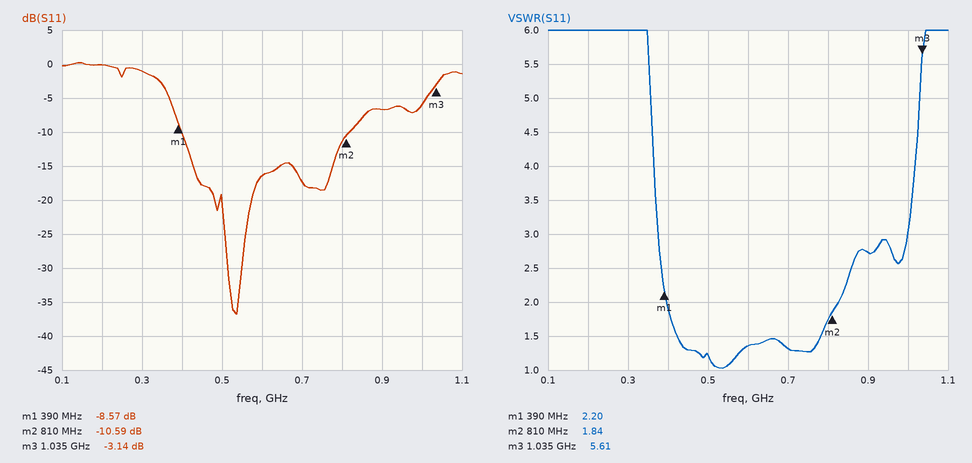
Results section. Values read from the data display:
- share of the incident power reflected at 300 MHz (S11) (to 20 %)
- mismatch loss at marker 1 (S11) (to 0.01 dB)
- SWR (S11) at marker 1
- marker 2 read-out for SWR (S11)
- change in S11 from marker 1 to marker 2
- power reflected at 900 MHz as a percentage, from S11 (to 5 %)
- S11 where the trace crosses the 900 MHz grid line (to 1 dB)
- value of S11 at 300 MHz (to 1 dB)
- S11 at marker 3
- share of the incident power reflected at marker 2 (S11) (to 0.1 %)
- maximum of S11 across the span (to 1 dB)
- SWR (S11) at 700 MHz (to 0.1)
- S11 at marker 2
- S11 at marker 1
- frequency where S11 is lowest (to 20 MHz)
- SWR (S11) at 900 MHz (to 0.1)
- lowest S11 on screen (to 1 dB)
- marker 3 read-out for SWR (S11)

80 %
0.65 dB
2.20
1.84
-2.02 dB
20 %
-7 dB
-1 dB
-3.14 dB
8.7 %
0 dB
1.3
-10.59 dB
-8.57 dB
540 MHz
2.7
-37 dB
5.61
